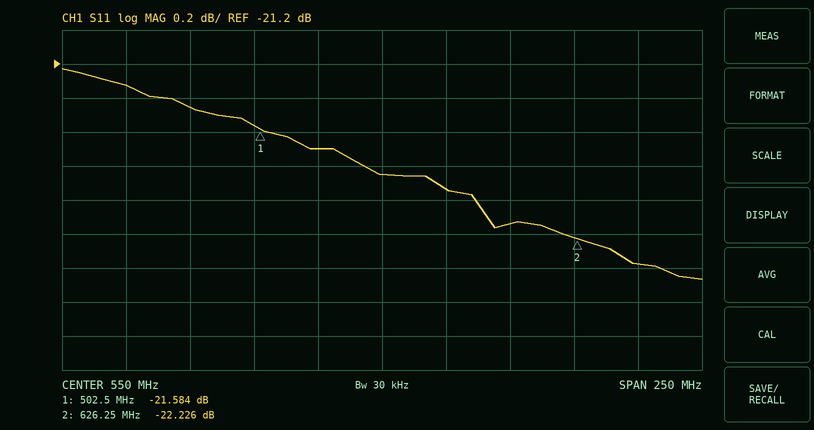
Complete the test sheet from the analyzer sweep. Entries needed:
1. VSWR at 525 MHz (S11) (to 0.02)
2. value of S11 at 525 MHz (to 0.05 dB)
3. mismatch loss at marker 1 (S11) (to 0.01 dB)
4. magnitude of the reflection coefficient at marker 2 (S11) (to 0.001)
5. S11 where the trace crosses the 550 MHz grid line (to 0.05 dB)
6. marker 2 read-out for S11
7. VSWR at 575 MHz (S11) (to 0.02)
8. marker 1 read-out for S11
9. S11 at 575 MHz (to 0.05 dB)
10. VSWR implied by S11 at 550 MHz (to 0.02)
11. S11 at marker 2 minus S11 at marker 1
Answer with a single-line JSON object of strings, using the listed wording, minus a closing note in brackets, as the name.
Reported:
{"VSWR at 525 MHz (S11)": "1.18", "value of S11 at 525 MHz": "-21.70 dB", "mismatch loss at marker 1 (S11)": "0.03 dB", "magnitude of the reflection coefficient at marker 2 (S11)": "0.077", "S11 where the trace crosses the 550 MHz grid line": "-21.85 dB", "marker 2 read-out for S11": "-22.226 dB", "VSWR at 575 MHz (S11)": "1.18", "marker 1 read-out for S11": "-21.584 dB", "S11 at 575 MHz": "-21.95 dB", "VSWR implied by S11 at 550 MHz": "1.18", "S11 at marker 2 minus S11 at marker 1": "-0.642 dB"}
